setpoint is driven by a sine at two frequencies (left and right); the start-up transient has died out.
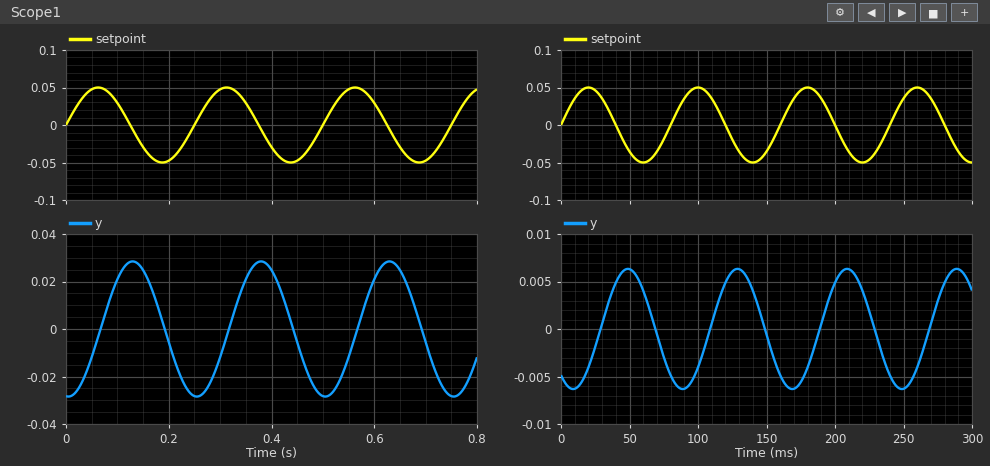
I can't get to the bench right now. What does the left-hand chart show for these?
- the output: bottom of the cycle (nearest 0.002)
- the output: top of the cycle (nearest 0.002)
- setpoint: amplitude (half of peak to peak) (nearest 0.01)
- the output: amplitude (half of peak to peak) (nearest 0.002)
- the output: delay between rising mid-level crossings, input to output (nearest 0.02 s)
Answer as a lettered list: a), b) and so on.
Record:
a) -0.028
b) 0.028
c) 0.05
d) 0.028
e) 0.06 s
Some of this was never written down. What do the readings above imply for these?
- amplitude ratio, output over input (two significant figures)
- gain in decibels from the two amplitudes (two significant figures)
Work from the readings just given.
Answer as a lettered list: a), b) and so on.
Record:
a) 0.56
b) -5.0 dB
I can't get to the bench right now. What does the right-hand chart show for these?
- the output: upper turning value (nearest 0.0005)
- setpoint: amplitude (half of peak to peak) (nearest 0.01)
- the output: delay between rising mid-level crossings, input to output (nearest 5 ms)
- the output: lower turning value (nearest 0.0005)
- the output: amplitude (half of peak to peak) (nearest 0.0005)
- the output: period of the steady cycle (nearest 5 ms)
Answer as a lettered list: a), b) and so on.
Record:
a) 0.0065
b) 0.05
c) 30 ms
d) -0.0065
e) 0.0065
f) 80 ms
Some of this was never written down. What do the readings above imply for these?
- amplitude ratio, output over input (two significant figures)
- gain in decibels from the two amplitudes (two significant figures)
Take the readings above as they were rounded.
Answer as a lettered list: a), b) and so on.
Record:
a) 0.13
b) -18 dB
